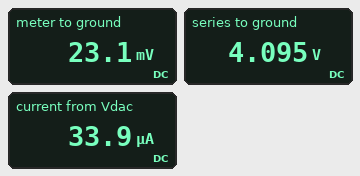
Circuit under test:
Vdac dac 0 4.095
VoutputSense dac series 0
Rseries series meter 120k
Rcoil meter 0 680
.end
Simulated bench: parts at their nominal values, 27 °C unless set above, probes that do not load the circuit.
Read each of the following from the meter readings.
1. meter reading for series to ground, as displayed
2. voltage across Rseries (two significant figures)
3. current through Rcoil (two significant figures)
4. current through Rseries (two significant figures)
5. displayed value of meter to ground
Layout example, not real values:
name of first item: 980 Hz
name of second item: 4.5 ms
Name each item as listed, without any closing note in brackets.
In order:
meter reading for series to ground, as displayed: 4.095 V
voltage across Rseries: 4.1 V
current through Rcoil: 34 µA
current through Rseries: 34 µA
displayed value of meter to ground: 23.1 mV
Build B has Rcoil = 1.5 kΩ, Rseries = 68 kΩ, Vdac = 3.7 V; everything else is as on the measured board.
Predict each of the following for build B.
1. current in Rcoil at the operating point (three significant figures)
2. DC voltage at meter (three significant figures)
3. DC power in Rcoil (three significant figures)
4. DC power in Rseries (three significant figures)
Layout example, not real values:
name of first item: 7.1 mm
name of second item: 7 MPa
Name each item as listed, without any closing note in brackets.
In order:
current in Rcoil at the operating point: 53.2 µA
DC voltage at meter: 79.9 mV
DC power in Rcoil: 4.25 µW
DC power in Rseries: 193 µW
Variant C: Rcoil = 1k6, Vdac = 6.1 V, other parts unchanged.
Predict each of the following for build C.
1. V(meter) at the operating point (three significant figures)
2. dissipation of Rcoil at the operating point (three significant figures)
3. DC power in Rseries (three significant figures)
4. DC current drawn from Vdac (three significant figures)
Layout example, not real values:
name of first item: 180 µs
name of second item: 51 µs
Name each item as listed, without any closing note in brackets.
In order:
V(meter) at the operating point: 80.3 mV
dissipation of Rcoil at the operating point: 4.03 µW
DC power in Rseries: 302 µW
DC current drawn from Vdac: 50.2 µA
